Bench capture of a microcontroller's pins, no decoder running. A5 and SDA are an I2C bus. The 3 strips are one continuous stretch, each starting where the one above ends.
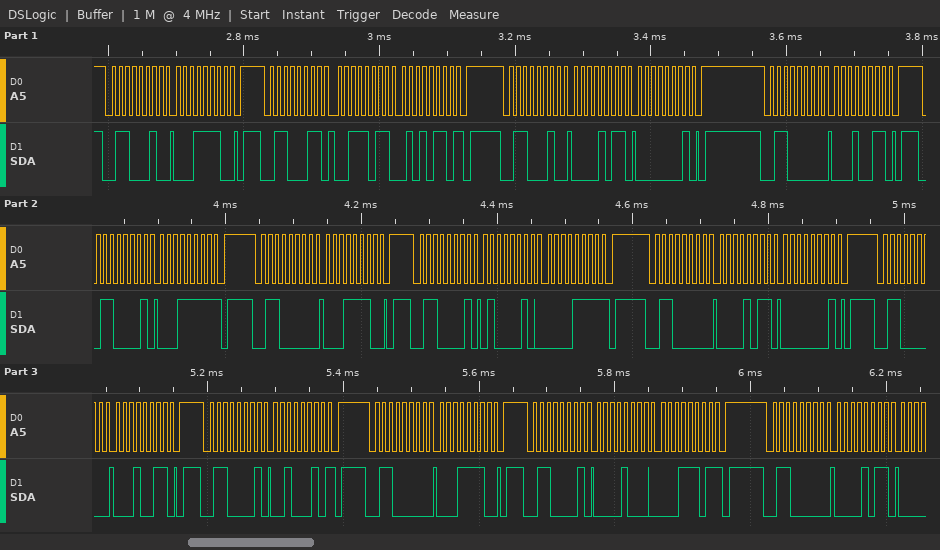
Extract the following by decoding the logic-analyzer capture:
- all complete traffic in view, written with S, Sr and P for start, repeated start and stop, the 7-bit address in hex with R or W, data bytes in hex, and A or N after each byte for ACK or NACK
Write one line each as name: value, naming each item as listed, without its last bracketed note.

all complete traffic in view, written with S, Sr and P for start, repeated start and stop, the 7-bit address in hex with R or W, data bytes in hex, and A or N after each byte for ACK or NACK: S 31W A 1E A P S 31R A 3B A 56 N P S 31W A 0B A 01 A P S 30W A 13 A P S 30R A 1F N P S 30W A 1E A P S 30R A 42 A 0F N P S 30W A 0B A 01 A P S 30W A 13 A P S 30R A 22 N P S 30W A 1E A P S 30R A 08 A 1D N P S 30W A 0B A
